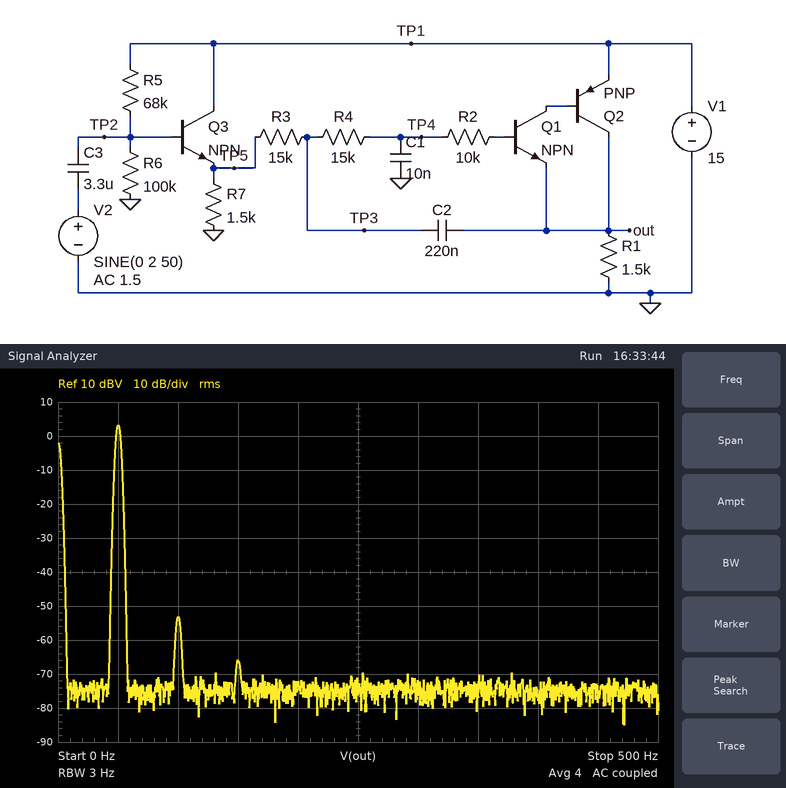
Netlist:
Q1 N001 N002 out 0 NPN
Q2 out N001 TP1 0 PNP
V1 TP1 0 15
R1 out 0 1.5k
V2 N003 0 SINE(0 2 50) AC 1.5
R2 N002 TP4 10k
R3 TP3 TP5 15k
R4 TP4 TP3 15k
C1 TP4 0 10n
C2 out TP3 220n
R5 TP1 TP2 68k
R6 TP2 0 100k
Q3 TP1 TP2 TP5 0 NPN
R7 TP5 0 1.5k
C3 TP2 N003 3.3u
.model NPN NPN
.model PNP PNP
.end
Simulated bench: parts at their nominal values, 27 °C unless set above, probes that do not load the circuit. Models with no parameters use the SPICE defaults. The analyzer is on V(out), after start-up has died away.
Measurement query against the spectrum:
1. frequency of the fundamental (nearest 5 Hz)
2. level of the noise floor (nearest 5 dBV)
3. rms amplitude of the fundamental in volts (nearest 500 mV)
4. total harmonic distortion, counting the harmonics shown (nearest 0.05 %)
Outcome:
50 Hz
-75 dBV
1.5 V
0.15 %
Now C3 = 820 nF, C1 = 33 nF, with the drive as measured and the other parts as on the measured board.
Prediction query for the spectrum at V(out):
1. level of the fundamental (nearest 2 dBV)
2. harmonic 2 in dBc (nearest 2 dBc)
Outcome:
4 dBV
-54 dBc
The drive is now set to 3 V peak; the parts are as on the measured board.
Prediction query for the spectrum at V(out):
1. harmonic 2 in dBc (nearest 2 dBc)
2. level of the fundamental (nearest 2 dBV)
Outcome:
-52 dBc
6 dBV
